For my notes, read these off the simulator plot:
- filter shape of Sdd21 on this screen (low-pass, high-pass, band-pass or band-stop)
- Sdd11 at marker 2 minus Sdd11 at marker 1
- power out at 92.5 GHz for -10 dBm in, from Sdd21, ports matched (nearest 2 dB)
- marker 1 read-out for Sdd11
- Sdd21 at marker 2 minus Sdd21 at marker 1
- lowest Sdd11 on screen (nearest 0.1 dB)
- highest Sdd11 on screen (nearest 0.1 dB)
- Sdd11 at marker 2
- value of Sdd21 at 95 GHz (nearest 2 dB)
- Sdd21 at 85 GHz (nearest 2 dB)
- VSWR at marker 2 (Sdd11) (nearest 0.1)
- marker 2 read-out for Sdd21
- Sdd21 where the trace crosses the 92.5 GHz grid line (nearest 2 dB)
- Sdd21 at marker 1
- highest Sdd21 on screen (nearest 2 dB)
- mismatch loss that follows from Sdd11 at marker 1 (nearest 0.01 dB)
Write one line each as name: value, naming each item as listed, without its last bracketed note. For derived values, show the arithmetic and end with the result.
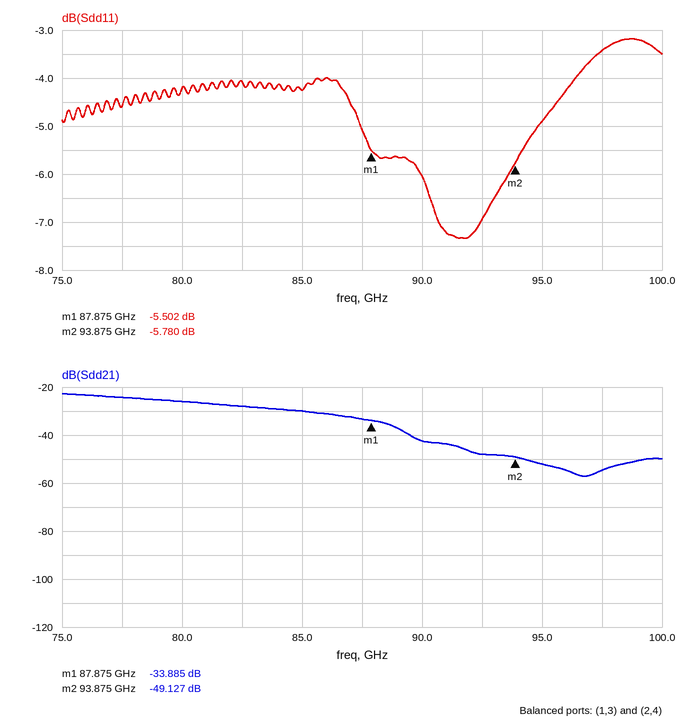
filter shape of Sdd21 on this screen: low-pass
Sdd11 at marker 2 minus Sdd11 at marker 1: -5.78 − (-5.502) = -0.278 dB
power out at 92.5 GHz for -10 dBm in, from Sdd21, ports matched: -10 dBm + (-48 dB) = -58 dBm
marker 1 read-out for Sdd11: -5.502 dB
Sdd21 at marker 2 minus Sdd21 at marker 1: -49.127 − (-33.885) = -15.242 dB
lowest Sdd11 on screen: -7.3 dB
highest Sdd11 on screen: -3.2 dB
Sdd11 at marker 2: -5.780 dB
value of Sdd21 at 95 GHz: -52 dB
Sdd21 at 85 GHz: -30 dB
VSWR at marker 2 (Sdd11): (1 + 0.5140)/(1 − 0.5140) ≈ 3.1
marker 2 read-out for Sdd21: -49.127 dB
Sdd21 where the trace crosses the 92.5 GHz grid line: -48 dB
Sdd21 at marker 1: -33.885 dB
highest Sdd21 on screen: -22 dB
mismatch loss that follows from Sdd11 at marker 1: −10 log10(1 − 10^(-5.502/10)) ≈ 1.44 dB
